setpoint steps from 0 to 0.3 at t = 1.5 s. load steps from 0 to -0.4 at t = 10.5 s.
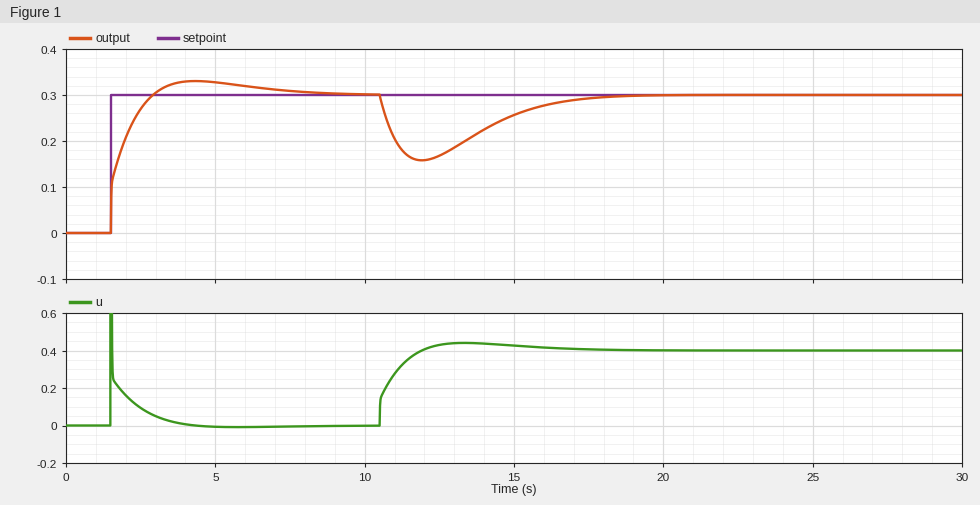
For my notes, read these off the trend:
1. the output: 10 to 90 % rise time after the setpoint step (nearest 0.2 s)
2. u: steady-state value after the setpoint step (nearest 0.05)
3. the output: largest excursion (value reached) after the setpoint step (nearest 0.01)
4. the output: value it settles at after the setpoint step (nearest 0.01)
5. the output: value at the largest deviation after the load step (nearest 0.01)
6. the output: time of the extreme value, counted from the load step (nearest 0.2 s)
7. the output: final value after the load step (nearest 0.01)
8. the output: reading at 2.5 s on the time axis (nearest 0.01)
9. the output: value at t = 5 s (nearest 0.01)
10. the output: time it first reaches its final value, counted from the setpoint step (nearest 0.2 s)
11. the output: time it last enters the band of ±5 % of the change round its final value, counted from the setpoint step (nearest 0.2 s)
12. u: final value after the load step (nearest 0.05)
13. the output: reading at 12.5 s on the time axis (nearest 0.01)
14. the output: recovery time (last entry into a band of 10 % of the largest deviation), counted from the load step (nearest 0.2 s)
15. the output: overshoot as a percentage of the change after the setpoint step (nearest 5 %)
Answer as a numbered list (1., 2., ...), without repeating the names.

1. 1.0 s
2. 0.00
3. 0.33
4. 0.30
5. 0.16
6. 1.4 s
7. 0.30
8. 0.27
9. 0.33
10. 1.4 s
11. 5.0 s
12. 0.40
13. 0.17
14. 6.2 s
15. 10 %
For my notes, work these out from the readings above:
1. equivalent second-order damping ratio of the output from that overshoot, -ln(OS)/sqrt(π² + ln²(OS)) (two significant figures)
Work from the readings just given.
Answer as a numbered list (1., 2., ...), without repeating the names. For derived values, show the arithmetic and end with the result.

1. ln(0.1) = -2.303; 2.303 / sqrt(9.870 + 5.302) = 0.59
